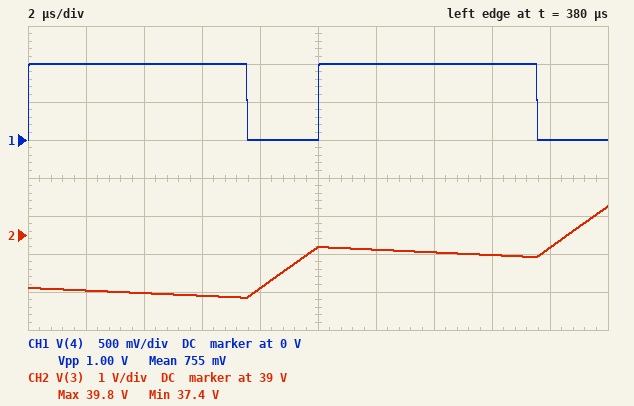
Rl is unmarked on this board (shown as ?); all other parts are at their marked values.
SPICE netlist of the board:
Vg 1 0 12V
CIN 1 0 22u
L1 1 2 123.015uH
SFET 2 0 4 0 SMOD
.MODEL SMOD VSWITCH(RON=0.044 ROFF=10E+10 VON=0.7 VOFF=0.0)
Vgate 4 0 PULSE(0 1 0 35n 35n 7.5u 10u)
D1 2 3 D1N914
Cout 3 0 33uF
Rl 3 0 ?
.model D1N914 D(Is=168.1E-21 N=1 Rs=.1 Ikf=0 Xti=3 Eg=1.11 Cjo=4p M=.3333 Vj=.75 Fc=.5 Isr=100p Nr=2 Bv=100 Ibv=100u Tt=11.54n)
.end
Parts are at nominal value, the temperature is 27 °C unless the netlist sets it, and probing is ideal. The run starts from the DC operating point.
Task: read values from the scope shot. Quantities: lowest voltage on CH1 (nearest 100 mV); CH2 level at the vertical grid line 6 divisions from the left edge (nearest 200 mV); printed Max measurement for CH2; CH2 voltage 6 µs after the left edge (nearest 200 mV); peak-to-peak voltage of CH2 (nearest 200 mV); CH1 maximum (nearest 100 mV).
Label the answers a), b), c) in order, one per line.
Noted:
a) 0 V
b) 38.6 V
c) 39.8 V
d) 37.4 V
e) 2.4 V
f) 1.0 V
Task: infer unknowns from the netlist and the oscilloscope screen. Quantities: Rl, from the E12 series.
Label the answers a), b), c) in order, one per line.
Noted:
a) 33 Ω
